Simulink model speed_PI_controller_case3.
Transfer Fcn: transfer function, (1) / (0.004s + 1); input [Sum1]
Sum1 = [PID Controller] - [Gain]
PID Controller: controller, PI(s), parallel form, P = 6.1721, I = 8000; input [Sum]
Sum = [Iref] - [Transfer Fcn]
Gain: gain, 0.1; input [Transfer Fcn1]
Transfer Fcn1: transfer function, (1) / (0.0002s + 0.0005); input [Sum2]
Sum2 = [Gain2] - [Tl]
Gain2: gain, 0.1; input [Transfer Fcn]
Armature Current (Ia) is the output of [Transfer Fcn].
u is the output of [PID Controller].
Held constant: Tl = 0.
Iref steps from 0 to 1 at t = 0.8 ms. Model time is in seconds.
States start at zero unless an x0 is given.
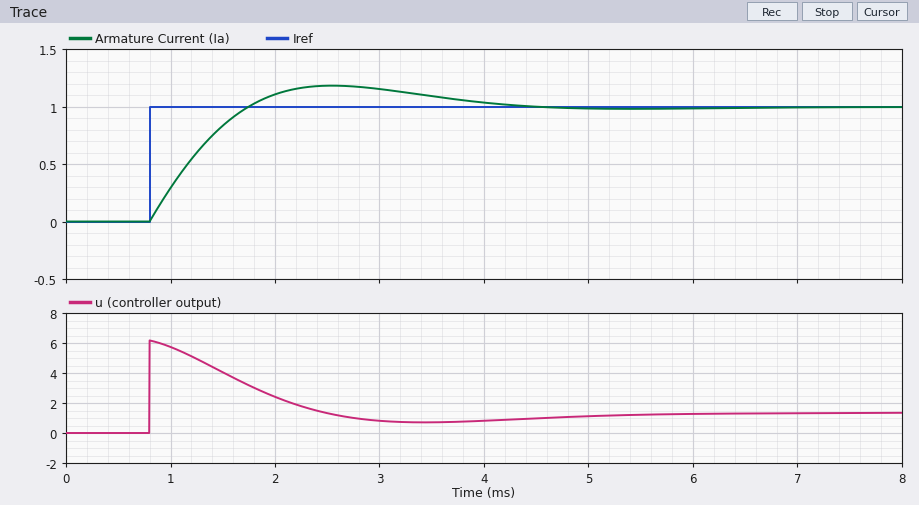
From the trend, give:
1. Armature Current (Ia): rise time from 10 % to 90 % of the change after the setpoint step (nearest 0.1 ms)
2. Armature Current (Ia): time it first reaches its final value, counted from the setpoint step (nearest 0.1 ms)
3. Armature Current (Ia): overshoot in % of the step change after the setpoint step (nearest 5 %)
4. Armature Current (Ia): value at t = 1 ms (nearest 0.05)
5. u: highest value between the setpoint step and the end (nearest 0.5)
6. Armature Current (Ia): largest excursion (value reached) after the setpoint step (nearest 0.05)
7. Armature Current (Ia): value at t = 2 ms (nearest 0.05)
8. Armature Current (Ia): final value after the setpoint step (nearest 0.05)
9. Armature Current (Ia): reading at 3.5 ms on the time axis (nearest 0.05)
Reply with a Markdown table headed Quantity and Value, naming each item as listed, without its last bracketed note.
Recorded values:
| Quantity | Value |
|---|---|
| Armature Current (Ia): rise time from 10 % to 90 % of the change after the setpoint step | 0.7 ms |
| Armature Current (Ia): time it first reaches its final value, counted from the setpoint step | 0.9 ms |
| Armature Current (Ia): overshoot in % of the step change after the setpoint step | 20 % |
| Armature Current (Ia): value at t = 1 ms | 0.30 |
| u: highest value between the setpoint step and the end | 6.0 |
| Armature Current (Ia): largest excursion (value reached) after the setpoint step | 1.20 |
| Armature Current (Ia): value at t = 2 ms | 1.10 |
| Armature Current (Ia): final value after the setpoint step | 1.00 |
| Armature Current (Ia): reading at 3.5 ms on the time axis | 1.10 |
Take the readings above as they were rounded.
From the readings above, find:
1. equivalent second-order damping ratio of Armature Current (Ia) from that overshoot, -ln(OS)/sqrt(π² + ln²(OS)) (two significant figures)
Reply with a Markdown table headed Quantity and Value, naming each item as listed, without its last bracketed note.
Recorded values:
| Quantity | Value |
|---|---|
| equivalent second-order damping ratio of Armature Current (Ia) from that overshoot, -ln(OS)/sqrt(π² + ln²(OS)) | 0.46 |
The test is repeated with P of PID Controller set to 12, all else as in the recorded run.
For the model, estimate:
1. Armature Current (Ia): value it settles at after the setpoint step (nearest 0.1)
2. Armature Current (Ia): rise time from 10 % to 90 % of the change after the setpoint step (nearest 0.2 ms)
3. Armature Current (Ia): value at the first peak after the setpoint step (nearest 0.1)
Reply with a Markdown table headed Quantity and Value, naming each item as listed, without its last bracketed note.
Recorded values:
| Quantity | Value |
|---|---|
| Armature Current (Ia): value it settles at after the setpoint step | 1.0 |
| Armature Current (Ia): rise time from 10 % to 90 % of the change after the setpoint step | 0.6 ms |
| Armature Current (Ia): value at the first peak after the setpoint step | 1.1 |
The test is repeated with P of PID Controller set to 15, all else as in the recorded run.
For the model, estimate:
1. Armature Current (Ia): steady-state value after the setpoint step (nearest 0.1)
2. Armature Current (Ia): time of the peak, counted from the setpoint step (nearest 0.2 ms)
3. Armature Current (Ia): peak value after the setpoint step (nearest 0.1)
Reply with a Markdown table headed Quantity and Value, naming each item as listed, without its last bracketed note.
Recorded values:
| Quantity | Value |
|---|---|
| Armature Current (Ia): steady-state value after the setpoint step | 1.0 |
| Armature Current (Ia): time of the peak, counted from the setpoint step | 1.4 ms |
| Armature Current (Ia): peak value after the setpoint step | 1.0 |
